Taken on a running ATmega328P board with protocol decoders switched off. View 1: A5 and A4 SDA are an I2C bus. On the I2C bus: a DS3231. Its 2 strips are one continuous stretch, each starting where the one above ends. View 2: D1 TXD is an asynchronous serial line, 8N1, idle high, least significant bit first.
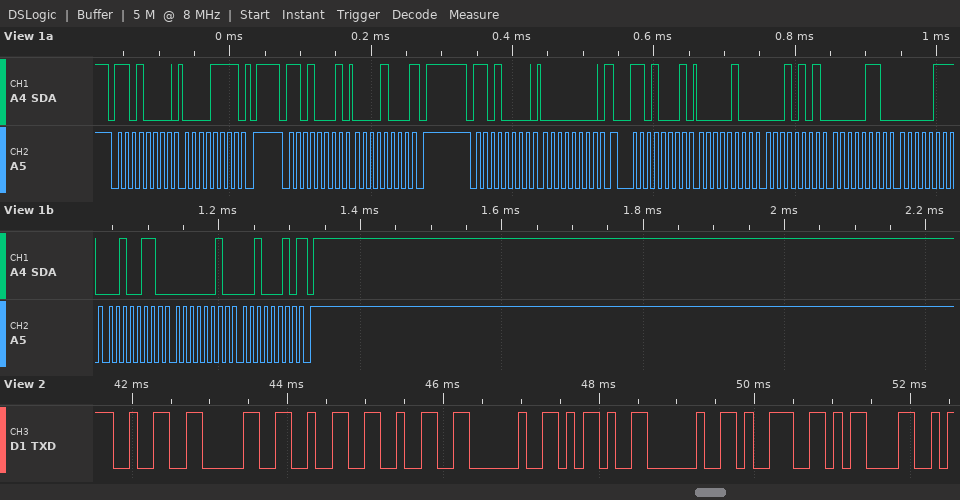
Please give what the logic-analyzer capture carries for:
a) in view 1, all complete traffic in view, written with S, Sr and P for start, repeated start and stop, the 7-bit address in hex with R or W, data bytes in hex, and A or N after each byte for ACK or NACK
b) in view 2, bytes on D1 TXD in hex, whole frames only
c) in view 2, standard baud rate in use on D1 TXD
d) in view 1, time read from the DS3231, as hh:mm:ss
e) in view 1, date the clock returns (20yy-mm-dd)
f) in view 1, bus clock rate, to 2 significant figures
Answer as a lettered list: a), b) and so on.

a) S 68W A 0F A P S 68R A 08 N P S 68W A 00 A Sr 68R A 04 A 15 A 06 A 07 A 26 A 02 A 22 N P
b) 32 30 32 32 20 2D 20 39 0D
c) 9600 baud
d) 06:15:04
e) 2022-02-26
f) 100 kHz
